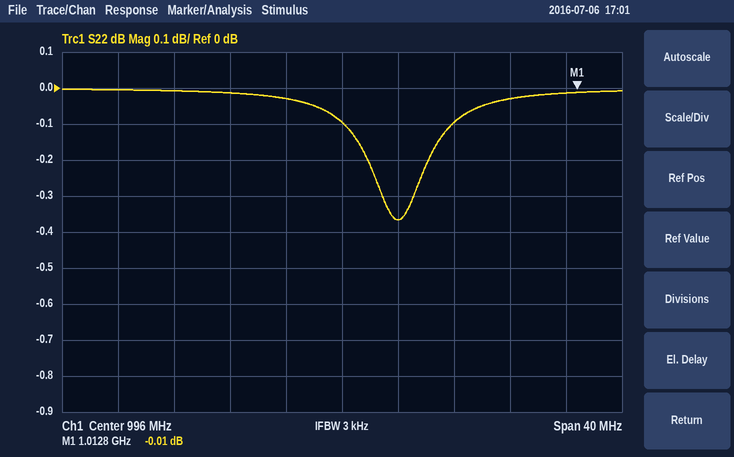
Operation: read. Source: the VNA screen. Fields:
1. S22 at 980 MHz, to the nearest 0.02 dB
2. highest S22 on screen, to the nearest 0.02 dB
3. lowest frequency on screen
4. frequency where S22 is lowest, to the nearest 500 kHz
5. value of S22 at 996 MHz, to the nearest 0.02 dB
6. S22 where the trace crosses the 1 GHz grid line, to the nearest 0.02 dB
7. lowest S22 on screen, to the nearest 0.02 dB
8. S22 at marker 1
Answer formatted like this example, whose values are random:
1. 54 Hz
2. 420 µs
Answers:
1. 0.00 dB
2. 0.00 dB
3. 976 MHz
4. 1.0000 GHz
5. -0.10 dB
6. -0.36 dB
7. -0.36 dB
8. -0.01 dB
